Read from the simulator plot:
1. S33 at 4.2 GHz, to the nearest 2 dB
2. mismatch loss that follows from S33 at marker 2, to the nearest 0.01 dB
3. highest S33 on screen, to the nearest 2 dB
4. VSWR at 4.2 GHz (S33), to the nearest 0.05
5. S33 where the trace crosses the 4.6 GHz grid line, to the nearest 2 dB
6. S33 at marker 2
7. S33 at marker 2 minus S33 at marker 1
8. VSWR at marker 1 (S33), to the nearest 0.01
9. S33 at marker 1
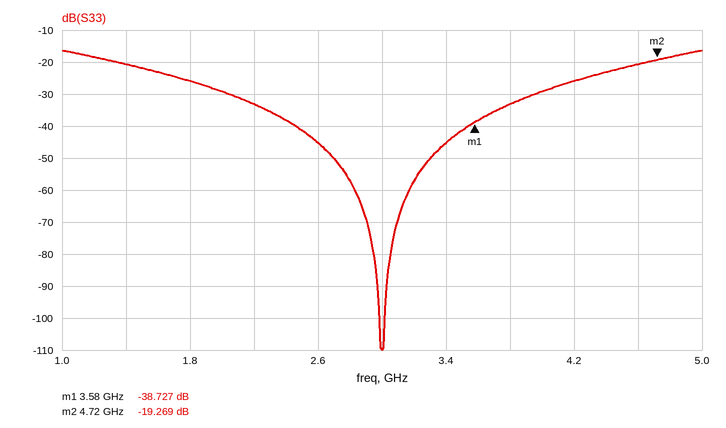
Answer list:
-26 dB
0.05 dB
-16 dB
1.10
-20 dB
-19.269 dB
19.458 dB
1.02
-38.727 dB
